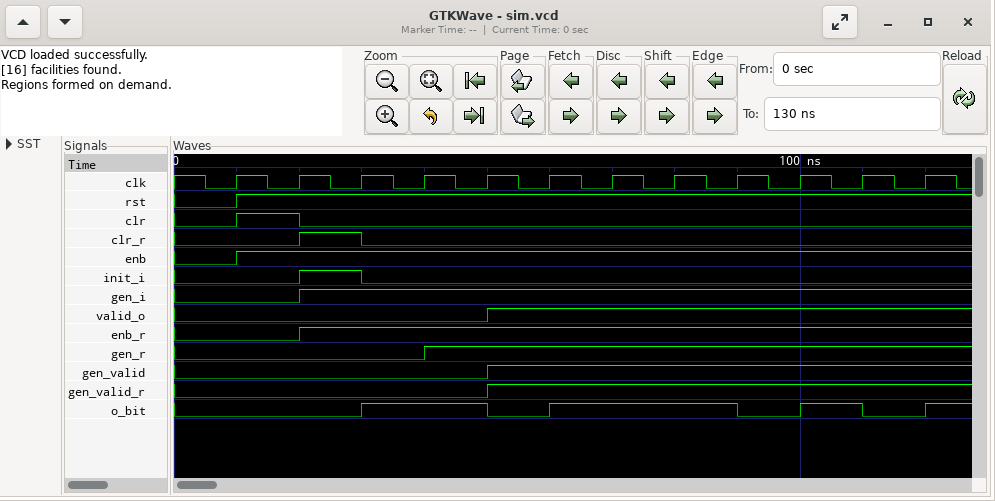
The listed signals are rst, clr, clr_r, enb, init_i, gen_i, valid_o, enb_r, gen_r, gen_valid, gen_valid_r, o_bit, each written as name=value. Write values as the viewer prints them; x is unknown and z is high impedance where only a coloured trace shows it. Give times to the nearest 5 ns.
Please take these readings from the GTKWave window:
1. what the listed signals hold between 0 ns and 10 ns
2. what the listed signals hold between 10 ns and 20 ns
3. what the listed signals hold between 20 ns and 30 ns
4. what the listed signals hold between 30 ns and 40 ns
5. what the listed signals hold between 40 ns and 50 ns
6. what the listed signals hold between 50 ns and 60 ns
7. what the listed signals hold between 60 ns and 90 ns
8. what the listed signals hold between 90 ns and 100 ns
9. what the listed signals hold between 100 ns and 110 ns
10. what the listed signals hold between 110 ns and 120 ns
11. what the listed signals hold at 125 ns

rst=0, clr=0, clr_r=0, enb=0, init_i=0, gen_i=0, valid_o=0, enb_r=0, gen_r=0, gen_valid=0, gen_valid_r=0, o_bit=0
rst=1, clr=1, clr_r=0, enb=1, init_i=0, gen_i=0, valid_o=0, enb_r=0, gen_r=0, gen_valid=0, gen_valid_r=0, o_bit=0
rst=1, clr=0, clr_r=1, enb=1, init_i=1, gen_i=1, valid_o=0, enb_r=1, gen_r=0, gen_valid=0, gen_valid_r=0, o_bit=0
rst=1, clr=0, clr_r=0, enb=1, init_i=0, gen_i=1, valid_o=0, enb_r=1, gen_r=0, gen_valid=0, gen_valid_r=0, o_bit=1
rst=1, clr=0, clr_r=0, enb=1, init_i=0, gen_i=1, valid_o=0, enb_r=1, gen_r=1, gen_valid=0, gen_valid_r=0, o_bit=1
rst=1, clr=0, clr_r=0, enb=1, init_i=0, gen_i=1, valid_o=1, enb_r=1, gen_r=1, gen_valid=1, gen_valid_r=1, o_bit=0
rst=1, clr=0, clr_r=0, enb=1, init_i=0, gen_i=1, valid_o=1, enb_r=1, gen_r=1, gen_valid=1, gen_valid_r=1, o_bit=1
rst=1, clr=0, clr_r=0, enb=1, init_i=0, gen_i=1, valid_o=1, enb_r=1, gen_r=1, gen_valid=1, gen_valid_r=1, o_bit=0
rst=1, clr=0, clr_r=0, enb=1, init_i=0, gen_i=1, valid_o=1, enb_r=1, gen_r=1, gen_valid=1, gen_valid_r=1, o_bit=1
rst=1, clr=0, clr_r=0, enb=1, init_i=0, gen_i=1, valid_o=1, enb_r=1, gen_r=1, gen_valid=1, gen_valid_r=1, o_bit=0
rst=1, clr=0, clr_r=0, enb=1, init_i=0, gen_i=1, valid_o=1, enb_r=1, gen_r=1, gen_valid=1, gen_valid_r=1, o_bit=1
